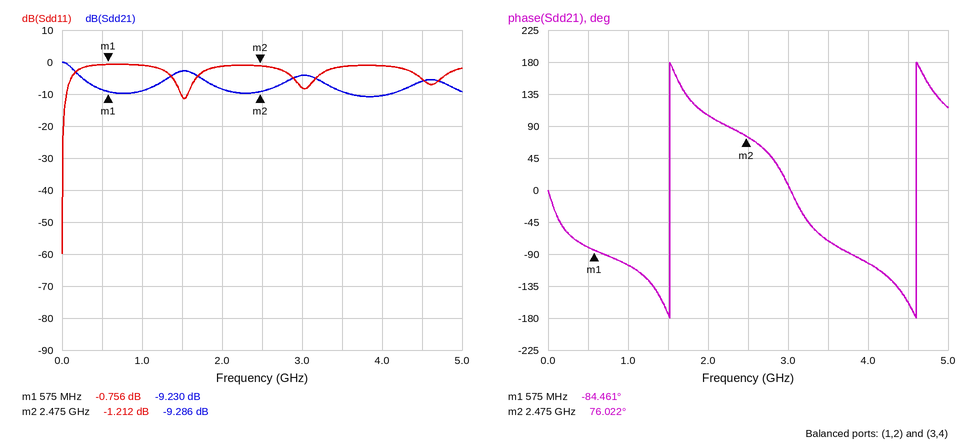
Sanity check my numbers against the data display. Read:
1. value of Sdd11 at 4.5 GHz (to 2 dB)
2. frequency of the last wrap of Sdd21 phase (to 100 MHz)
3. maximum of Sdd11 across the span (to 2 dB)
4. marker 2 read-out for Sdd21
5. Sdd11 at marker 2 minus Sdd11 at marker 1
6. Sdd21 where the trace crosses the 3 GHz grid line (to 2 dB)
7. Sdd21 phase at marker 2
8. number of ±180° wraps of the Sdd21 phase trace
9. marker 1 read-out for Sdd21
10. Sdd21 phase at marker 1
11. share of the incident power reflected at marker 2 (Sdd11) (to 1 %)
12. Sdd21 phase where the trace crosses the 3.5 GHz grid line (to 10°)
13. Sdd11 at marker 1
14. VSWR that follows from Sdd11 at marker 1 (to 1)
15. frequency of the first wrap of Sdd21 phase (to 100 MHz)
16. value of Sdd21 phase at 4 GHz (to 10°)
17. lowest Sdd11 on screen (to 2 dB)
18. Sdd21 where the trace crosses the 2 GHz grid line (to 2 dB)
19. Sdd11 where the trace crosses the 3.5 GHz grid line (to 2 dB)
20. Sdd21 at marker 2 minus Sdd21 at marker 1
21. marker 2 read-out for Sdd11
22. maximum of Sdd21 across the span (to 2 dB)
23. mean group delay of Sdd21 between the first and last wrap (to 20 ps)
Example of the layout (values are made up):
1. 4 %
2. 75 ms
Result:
1. -6 dB
2. 4.6 GHz
3. 0 dB
4. -9.286 dB
5. -0.456 dB
6. -4 dB
7. 76.022°
8. 2
9. -9.230 dB
10. -84.461°
11. 76 %
12. -70°
13. -0.756 dB
14. 23
15. 1.5 GHz
16. -100°
17. -60 dB
18. -8 dB
19. -2 dB
20. -0.056 dB
21. -1.212 dB
22. 0 dB
23. 320 ps
